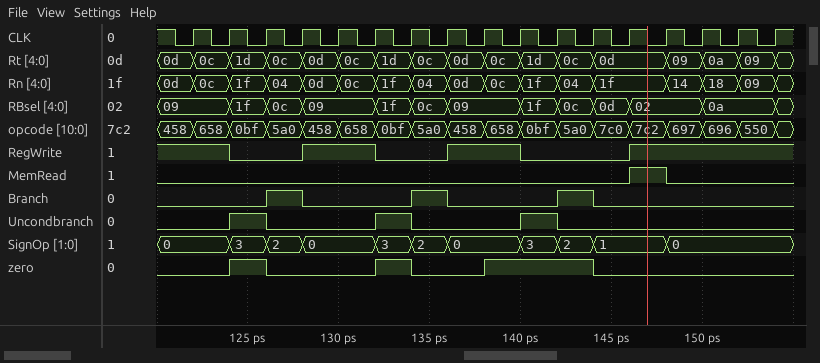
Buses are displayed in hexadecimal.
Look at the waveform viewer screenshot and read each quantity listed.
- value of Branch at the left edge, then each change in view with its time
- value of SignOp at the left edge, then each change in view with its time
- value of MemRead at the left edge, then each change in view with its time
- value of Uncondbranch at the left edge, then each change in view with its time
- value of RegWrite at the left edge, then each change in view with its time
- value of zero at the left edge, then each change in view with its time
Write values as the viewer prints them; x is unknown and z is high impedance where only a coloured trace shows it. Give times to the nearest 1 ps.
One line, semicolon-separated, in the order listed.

0, 1 at 126 ps, 0 at 128 ps, 1 at 134 ps, 0 at 136 ps, 1 at 142 ps, 0 at 144 ps; 0, 3 at 124 ps, 2 at 126 ps, 0 at 128 ps, 3 at 132 ps, 2 at 134 ps, 0 at 136 ps, 3 at 140 ps, 2 at 142 ps, 1 at 144 ps, 0 at 148 ps; 0, 1 at 146 ps, 0 at 148 ps; 0, 1 at 124 ps, 0 at 126 ps, 1 at 132 ps, 0 at 134 ps, 1 at 140 ps, 0 at 142 ps; 1, 0 at 124 ps, 1 at 128 ps, 0 at 132 ps, 1 at 136 ps, 0 at 140 ps, 1 at 146 ps; 0, 1 at 124 ps, 0 at 126 ps, 1 at 132 ps, 0 at 134 ps, 1 at 138 ps, 0 at 144 ps
